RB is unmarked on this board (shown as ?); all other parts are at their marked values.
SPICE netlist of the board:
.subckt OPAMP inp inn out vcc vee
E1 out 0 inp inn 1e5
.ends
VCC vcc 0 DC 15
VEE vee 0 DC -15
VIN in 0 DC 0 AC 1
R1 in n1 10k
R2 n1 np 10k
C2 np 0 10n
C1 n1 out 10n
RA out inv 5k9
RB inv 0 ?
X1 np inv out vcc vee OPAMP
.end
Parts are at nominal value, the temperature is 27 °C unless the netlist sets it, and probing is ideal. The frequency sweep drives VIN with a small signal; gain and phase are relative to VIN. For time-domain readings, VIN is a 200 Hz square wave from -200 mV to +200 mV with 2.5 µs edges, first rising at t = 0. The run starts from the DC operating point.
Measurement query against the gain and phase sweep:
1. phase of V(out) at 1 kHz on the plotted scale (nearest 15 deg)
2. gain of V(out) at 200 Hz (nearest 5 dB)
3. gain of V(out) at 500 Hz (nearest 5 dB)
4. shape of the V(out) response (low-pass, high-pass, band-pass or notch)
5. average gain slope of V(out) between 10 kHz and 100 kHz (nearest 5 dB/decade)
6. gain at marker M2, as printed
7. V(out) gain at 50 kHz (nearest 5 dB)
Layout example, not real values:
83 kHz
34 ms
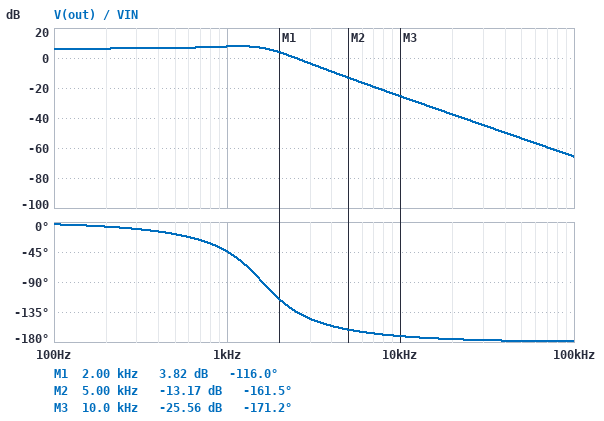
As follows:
-45 deg
5 dB
5 dB
low-pass
-40 dB/decade
-13.17 dB
-55 dB
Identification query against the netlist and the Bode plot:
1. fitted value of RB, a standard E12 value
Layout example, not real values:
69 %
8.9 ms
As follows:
5.6 kΩ
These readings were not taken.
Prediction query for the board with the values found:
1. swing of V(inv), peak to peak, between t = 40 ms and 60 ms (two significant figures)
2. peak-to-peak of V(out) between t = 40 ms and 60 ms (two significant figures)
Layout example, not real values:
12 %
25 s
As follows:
550 mV
1.1 V
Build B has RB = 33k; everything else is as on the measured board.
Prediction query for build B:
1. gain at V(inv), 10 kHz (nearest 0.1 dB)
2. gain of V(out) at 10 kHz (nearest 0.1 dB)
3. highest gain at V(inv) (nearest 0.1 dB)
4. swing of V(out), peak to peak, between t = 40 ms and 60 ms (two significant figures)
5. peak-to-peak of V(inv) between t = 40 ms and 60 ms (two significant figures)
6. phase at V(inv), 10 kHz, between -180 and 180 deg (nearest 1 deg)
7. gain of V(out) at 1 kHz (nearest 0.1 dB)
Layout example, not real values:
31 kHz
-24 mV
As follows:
-32.1 dB
-30.6 dB
0 dB
470 mV
400 mV
-163 deg
-0.8 dB
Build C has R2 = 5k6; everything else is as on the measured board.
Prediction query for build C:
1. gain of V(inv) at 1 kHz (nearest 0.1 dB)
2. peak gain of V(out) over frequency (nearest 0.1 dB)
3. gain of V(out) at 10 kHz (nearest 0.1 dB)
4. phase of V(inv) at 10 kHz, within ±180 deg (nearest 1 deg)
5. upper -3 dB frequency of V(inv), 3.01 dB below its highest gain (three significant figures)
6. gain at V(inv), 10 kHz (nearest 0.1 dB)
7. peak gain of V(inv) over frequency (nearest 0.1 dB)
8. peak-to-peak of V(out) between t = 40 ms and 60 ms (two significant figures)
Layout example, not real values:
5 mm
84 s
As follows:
1.5 dB
10.2 dB
-20.3 dB
-171 deg
2.52 kHz
-26.6 dB
3.9 dB
1.4 V
